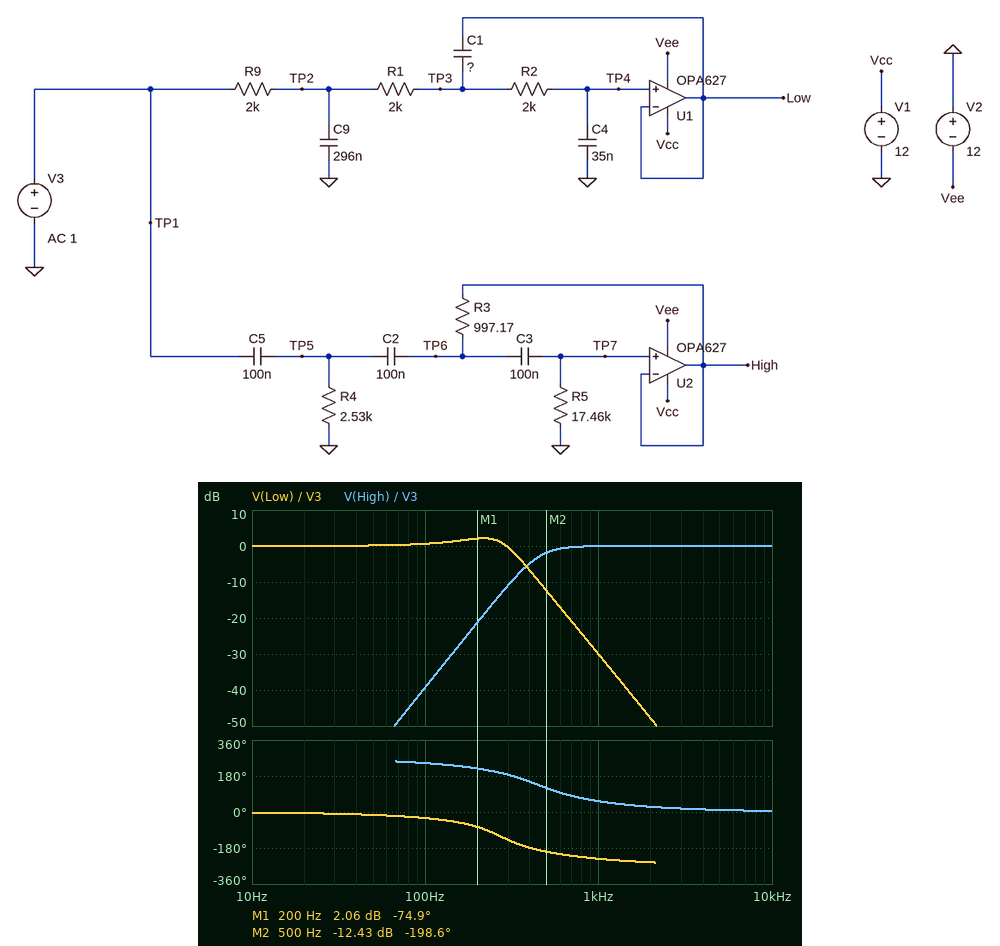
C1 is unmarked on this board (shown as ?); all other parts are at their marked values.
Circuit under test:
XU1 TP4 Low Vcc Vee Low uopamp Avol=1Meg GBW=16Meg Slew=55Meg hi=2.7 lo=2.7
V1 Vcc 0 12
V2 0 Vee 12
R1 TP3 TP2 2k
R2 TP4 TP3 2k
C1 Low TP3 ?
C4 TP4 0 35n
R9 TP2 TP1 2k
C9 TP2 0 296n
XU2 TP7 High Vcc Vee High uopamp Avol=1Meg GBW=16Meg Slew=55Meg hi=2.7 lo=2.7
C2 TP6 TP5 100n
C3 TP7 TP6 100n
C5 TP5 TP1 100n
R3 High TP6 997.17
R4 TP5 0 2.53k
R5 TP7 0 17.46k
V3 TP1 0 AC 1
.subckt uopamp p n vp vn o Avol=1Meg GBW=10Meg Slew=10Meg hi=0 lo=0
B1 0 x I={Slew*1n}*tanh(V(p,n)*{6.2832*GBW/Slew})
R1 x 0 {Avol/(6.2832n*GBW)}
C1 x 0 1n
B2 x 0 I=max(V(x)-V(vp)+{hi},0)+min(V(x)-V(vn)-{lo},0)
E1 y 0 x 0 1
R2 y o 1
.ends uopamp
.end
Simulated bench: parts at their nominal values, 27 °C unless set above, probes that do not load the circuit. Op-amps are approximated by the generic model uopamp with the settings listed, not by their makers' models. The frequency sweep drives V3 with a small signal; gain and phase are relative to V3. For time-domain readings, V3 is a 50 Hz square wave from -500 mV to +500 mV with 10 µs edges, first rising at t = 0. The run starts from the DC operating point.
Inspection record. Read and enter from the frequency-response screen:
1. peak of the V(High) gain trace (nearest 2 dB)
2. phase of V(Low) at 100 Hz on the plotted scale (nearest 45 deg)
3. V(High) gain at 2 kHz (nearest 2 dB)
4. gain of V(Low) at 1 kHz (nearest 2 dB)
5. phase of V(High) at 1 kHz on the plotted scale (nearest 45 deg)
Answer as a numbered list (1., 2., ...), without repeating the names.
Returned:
1. 0 dB
2. -45 deg
3. 0 dB
4. -30 dB
5. 45 deg
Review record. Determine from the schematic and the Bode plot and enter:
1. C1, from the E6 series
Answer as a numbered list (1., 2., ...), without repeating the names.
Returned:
1. 1.5 µF
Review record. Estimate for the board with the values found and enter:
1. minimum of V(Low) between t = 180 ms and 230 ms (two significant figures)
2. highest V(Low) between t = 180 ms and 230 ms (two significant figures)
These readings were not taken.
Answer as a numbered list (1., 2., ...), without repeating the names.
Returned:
1. -730 mV
2. 730 mV
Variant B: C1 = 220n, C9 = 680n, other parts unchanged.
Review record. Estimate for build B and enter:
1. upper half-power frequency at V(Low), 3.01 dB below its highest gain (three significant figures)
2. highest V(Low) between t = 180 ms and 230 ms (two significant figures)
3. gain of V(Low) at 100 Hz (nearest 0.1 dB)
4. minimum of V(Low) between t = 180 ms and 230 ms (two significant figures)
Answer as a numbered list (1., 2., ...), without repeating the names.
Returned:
1. 115 Hz
2. 500 mV
3. -2.5 dB
4. -500 mV
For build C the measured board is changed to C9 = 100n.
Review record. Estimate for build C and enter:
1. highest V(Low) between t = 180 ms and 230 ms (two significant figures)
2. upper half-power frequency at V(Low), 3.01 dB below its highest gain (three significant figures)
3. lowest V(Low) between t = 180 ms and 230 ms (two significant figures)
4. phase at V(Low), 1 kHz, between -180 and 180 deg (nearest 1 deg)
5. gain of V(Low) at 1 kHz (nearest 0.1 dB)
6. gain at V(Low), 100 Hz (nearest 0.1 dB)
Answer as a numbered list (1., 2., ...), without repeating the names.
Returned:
1. 960 mV
2. 286 Hz
3. -960 mV
4. 155 deg
5. -25.3 dB
6. 1.3 dB
